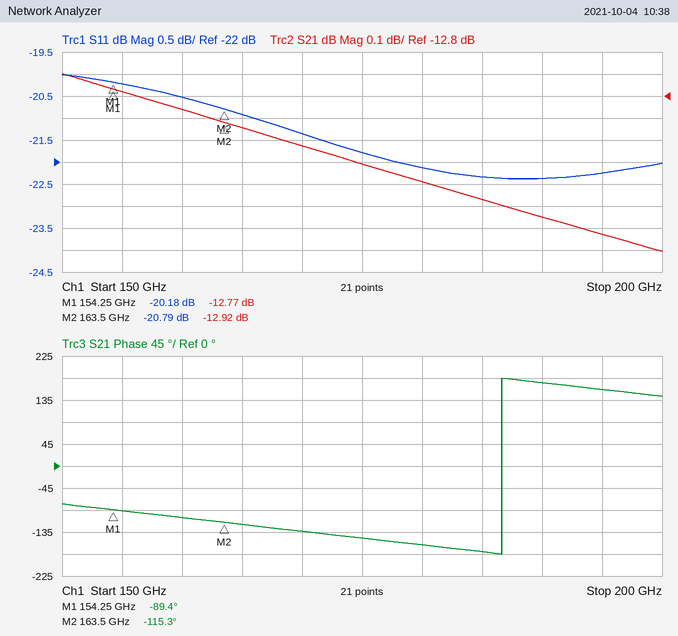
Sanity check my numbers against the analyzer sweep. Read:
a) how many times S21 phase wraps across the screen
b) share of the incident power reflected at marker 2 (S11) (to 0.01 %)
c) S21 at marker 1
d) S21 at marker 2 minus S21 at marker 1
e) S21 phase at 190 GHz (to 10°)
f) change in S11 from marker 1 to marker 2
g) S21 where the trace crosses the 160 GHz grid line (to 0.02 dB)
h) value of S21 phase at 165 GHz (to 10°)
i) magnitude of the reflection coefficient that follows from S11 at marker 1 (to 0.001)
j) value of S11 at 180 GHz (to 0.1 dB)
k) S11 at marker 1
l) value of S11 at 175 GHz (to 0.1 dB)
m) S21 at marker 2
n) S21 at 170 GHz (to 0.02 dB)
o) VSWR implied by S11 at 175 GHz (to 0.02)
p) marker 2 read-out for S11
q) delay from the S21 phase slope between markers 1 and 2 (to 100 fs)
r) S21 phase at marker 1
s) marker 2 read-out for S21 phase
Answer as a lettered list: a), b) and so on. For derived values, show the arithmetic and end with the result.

a) 1
b) 10^(-20.79/10) ≈ 0.83 %
c) -12.77 dB
d) -12.92 − (-12.77) = -0.15 dB
e) 170°
f) -20.79 − (-20.18) = -0.61 dB
g) -12.86 dB
h) -120°
i) 10^(-20.18/20) ≈ 0.098
j) -22.1 dB
k) -20.18 dB
l) -21.8 dB
m) -12.92 dB
n) -13.02 dB
o) |Γ| = 10^(-21.8/20) = 0.0813; VSWR = (1 + 0.0813)/(1 − 0.0813) ≈ 1.18
p) -20.79 dB
q) −(-115.3° − (-89.4°))/(360° × 9.25 GHz) ≈ 7.8 ps
r) -89.4°
s) -115.3°
